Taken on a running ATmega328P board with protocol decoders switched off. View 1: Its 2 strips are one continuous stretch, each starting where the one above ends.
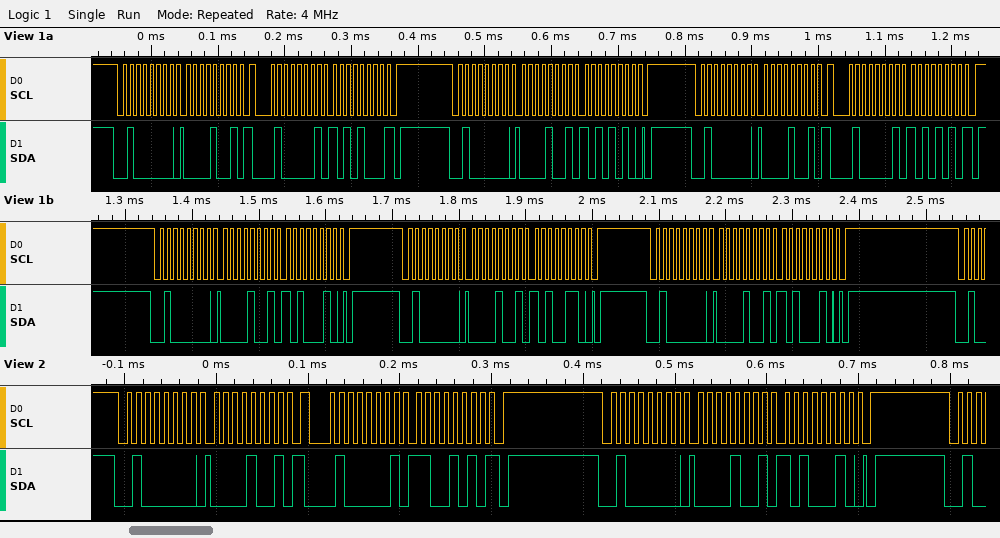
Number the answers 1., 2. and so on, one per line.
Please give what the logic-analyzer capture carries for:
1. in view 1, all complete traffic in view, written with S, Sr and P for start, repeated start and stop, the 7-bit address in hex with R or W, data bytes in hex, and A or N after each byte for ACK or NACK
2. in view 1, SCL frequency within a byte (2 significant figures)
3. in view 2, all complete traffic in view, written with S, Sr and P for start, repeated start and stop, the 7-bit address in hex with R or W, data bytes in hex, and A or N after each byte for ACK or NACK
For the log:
1. S 20W A 09 A Sr 20R A A8 N P S 20W A 09 A AA A P S 20W A 09 A Sr 20R A AA N P S 20W A 09 A A2 A P S 20W A 09 A A6 A P S 20W A 09 A A2 A P
2. 100 kHz
3. S 20W A 09 A Sr 20R A CA N P S 20W A 09 A A2 A P
